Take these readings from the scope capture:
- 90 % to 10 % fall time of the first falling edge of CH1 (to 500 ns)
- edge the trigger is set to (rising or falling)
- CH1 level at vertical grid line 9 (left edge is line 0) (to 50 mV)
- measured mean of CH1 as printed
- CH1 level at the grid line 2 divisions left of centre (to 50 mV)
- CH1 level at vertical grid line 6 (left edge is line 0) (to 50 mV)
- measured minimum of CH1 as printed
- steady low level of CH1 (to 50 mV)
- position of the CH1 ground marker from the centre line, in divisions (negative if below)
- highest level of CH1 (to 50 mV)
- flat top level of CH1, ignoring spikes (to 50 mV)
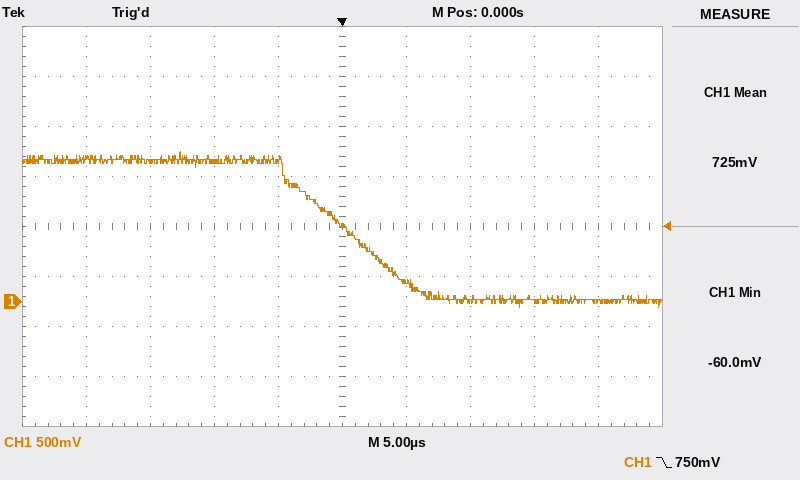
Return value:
10.0 µs
falling
0 mV
725 mV
1.40 V
200 mV
-60.0 mV
0 mV
-1.5 div
1.50 V
1.40 V
